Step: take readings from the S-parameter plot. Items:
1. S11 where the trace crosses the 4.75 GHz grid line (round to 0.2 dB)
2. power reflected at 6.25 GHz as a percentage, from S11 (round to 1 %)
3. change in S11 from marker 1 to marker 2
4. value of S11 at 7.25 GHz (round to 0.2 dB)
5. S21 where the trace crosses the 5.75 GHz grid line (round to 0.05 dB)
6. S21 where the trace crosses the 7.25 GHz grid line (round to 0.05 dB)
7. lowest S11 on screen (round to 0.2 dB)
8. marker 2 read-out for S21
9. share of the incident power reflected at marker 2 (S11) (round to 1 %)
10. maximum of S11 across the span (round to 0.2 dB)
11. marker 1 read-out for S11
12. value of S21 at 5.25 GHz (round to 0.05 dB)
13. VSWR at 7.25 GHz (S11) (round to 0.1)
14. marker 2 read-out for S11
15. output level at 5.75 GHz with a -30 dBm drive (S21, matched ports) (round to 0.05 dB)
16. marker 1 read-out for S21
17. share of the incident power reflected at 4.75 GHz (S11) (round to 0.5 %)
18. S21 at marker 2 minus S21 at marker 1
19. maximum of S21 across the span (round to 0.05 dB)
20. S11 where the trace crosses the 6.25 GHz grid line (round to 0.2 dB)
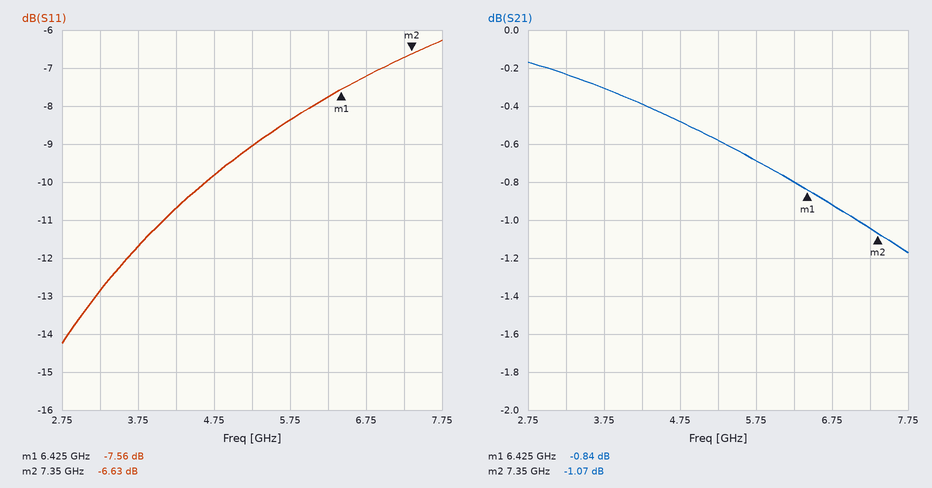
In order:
-9.8 dB
17 %
0.93 dB
-6.8 dB
-0.70 dB
-1.05 dB
-14.2 dB
-1.07 dB
22 %
-6.2 dB
-7.56 dB
-0.60 dB
2.7
-6.63 dB
-30.70 dBm
-0.84 dB
10.5 %
-0.23 dB
-0.15 dB
-7.8 dB
